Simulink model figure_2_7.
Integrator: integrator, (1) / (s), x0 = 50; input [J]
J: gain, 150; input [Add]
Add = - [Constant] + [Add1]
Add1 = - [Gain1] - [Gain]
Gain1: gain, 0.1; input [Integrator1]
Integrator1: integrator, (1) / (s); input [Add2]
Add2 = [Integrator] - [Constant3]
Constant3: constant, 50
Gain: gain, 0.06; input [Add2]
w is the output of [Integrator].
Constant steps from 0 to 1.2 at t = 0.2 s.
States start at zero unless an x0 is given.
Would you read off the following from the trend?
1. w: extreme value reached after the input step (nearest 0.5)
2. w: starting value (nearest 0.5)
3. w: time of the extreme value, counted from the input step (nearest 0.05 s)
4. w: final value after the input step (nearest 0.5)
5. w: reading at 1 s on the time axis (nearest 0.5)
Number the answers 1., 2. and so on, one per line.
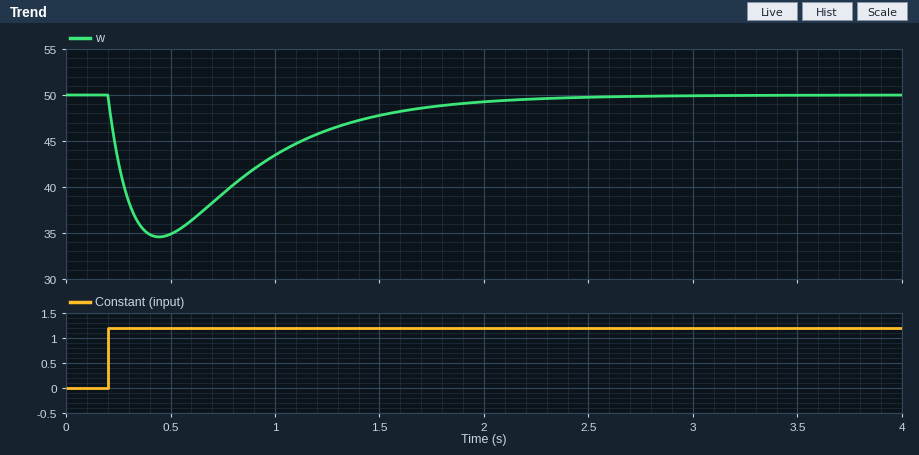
1. 34.5
2. 50.0
3. 0.25 s
4. 50.0
5. 43.5
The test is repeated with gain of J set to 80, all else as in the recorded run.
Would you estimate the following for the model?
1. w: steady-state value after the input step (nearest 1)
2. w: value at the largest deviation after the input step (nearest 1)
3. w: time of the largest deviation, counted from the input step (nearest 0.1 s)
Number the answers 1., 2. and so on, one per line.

1. 50
2. 36
3. 0.4 s
